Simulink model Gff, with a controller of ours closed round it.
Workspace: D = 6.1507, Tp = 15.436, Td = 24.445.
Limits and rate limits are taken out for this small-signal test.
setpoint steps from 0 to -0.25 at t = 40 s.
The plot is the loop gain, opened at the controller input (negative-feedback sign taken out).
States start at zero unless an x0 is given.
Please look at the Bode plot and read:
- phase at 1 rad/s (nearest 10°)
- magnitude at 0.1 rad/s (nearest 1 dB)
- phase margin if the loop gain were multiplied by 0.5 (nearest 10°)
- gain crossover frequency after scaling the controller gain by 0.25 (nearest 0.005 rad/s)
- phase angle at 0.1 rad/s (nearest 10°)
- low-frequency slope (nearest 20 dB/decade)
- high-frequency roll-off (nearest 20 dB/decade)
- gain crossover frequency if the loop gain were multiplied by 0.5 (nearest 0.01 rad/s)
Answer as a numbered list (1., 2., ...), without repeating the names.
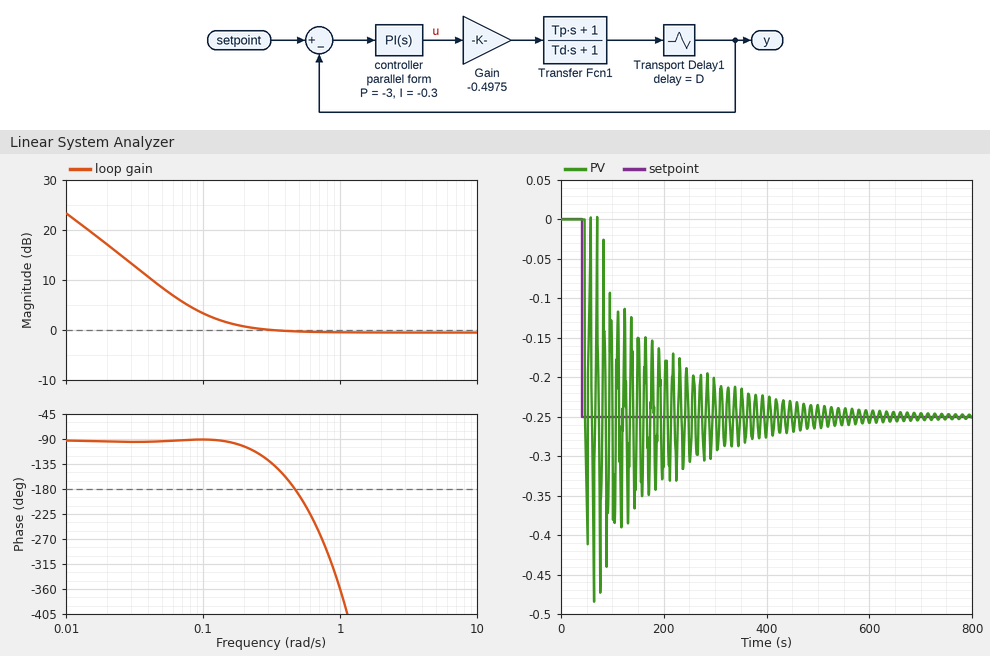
1. -360°
2. 3 dB
3. 90°
4. 0.035 rad/s
5. -90°
6. -20 dB/decade
7. 0 dB/decade
8. 0.07 rad/s
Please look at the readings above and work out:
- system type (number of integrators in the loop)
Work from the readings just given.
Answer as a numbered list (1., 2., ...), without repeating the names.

1. 1
